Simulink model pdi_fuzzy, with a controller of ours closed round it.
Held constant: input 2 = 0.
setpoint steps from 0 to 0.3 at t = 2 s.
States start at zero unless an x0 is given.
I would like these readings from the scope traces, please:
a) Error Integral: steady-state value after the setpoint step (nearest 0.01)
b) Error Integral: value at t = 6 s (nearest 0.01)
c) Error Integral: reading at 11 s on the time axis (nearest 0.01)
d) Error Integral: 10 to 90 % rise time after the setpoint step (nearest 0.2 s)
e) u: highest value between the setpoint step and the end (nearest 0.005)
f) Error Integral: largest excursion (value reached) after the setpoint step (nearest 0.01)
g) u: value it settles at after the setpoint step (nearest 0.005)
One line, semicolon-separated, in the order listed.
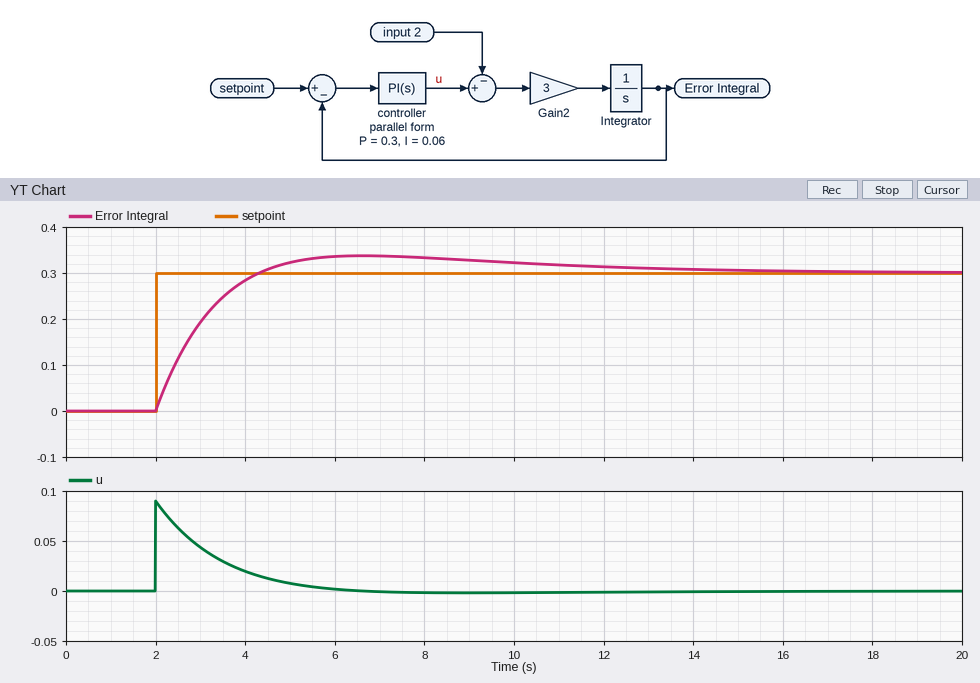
0.30; 0.34; 0.32; 1.6 s; 0.090; 0.34; 0.000
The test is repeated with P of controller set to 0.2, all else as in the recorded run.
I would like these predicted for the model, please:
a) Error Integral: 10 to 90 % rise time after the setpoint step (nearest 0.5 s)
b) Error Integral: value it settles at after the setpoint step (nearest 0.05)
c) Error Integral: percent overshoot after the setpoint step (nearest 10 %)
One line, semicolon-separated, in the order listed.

2.0 s; 0.30; 20 %
